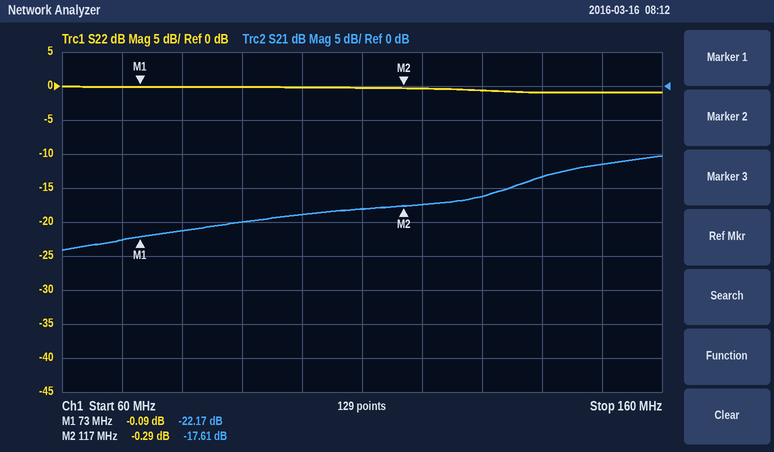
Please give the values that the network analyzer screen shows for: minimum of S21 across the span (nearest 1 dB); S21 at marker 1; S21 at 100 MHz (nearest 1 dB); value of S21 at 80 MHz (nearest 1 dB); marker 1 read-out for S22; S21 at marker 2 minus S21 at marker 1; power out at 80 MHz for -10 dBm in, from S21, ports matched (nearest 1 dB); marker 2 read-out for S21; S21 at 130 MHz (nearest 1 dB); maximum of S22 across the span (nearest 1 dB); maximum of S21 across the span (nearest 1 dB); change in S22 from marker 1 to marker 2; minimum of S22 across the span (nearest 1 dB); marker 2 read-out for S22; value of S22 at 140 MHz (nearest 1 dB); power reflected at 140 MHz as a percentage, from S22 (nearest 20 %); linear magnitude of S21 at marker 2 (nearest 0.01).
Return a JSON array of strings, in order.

["-24 dB", "-22.17 dB", "-19 dB", "-21 dB", "-0.09 dB", "4.56 dB", "-31 dBm", "-17.61 dB", "-16 dB", "0 dB", "-10 dB", "-0.20 dB", "-1 dB", "-0.29 dB", "-1 dB", "80 %", "0.13"]
